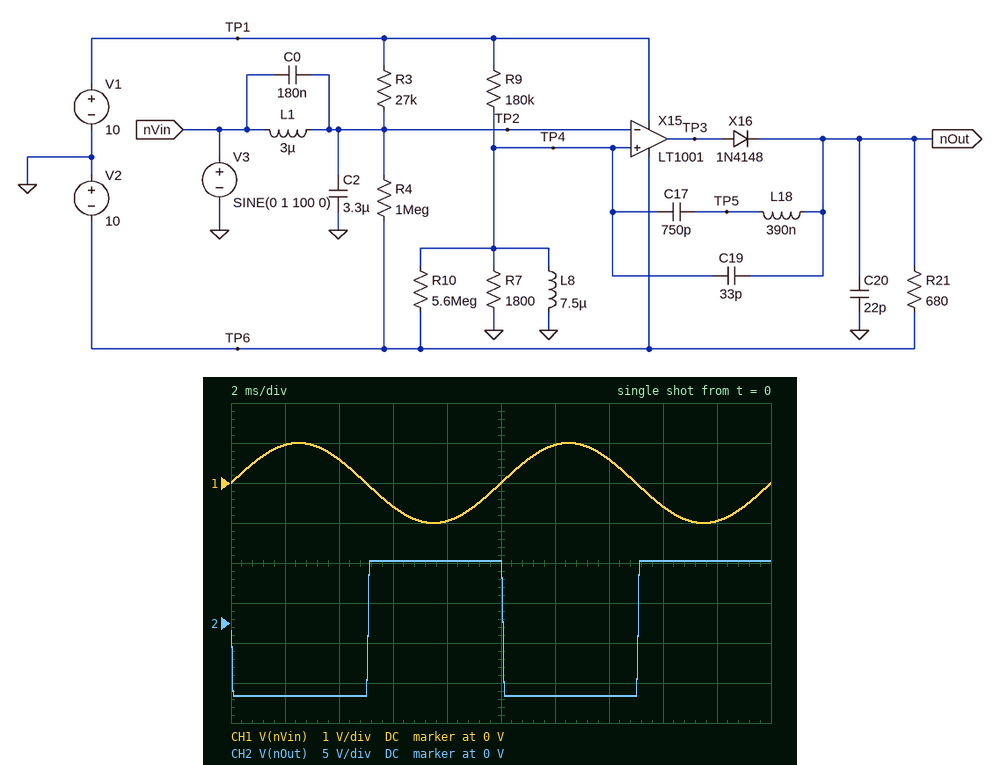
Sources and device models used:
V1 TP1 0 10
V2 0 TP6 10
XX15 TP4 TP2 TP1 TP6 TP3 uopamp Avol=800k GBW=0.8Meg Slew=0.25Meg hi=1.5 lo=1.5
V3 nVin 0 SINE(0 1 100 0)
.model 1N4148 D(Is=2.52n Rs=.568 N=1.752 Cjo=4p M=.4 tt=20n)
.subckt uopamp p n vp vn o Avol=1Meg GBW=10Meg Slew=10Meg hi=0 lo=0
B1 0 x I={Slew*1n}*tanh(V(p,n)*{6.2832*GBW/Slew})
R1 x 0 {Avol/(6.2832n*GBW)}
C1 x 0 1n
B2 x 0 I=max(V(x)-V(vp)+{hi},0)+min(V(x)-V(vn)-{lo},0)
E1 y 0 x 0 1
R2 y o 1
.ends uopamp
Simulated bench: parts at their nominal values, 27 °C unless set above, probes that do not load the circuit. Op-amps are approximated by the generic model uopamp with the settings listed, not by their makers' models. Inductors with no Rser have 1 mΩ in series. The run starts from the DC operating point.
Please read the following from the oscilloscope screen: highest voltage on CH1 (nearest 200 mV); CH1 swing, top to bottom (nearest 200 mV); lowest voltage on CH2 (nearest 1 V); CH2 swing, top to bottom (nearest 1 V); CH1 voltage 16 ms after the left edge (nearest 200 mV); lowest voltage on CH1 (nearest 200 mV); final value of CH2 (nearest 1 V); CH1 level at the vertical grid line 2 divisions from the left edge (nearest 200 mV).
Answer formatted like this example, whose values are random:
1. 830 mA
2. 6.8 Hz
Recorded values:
1. 1.0 V
2. 2.0 V
3. -9 V
4. 17 V
5. -600 mV
6. -1.0 V
7. 8 V
8. 600 mV
